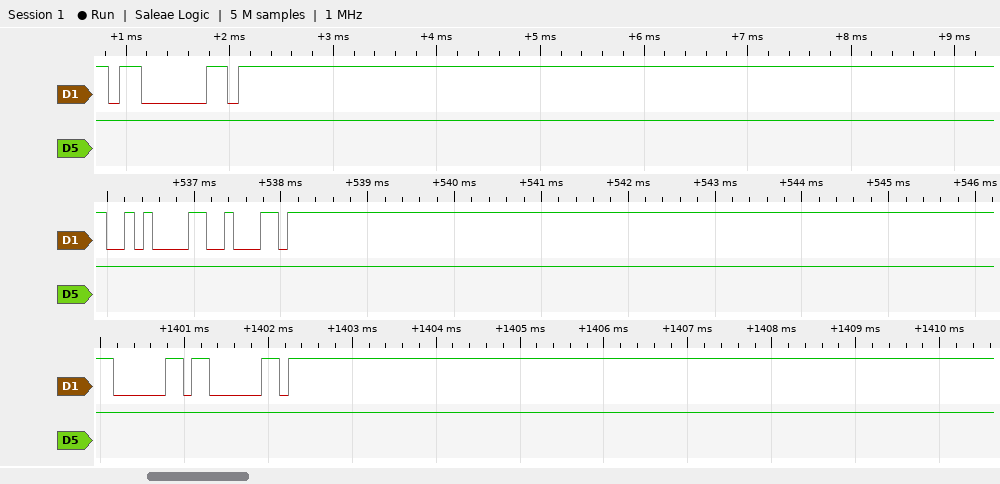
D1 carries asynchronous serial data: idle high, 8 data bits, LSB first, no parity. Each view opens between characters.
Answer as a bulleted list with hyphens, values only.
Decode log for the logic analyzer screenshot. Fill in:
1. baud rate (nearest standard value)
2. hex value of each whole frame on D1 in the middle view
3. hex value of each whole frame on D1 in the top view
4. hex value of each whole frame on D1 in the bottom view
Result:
- 9600 baud
- 0A, 62
- 03, FF
- 60, 60
